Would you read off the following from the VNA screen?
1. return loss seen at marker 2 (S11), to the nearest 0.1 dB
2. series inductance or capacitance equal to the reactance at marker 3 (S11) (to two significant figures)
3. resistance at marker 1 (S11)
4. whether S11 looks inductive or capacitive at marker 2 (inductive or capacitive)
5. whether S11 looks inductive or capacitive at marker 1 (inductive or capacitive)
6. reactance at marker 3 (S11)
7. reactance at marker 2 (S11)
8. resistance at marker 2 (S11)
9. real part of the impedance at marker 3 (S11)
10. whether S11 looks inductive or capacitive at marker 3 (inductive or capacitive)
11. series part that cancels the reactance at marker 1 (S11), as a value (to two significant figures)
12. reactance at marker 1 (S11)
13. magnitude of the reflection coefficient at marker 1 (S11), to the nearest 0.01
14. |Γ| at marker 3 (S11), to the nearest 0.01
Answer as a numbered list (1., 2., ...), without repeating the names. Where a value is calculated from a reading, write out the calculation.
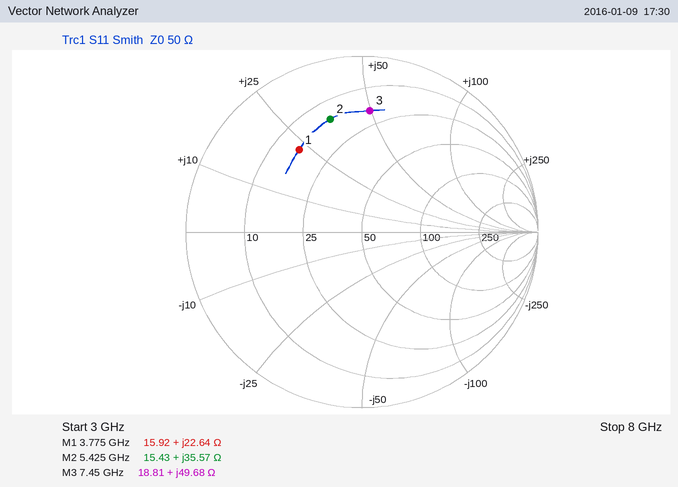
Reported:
1. 3.5 dB
2. L = 49.68 Ω/(2π × 7.45 GHz) ≈ 1.1 nH
3. 15.92 Ω
4. inductive
5. inductive
6. +49.68 Ω
7. +35.57 Ω
8. 15.43 Ω
9. 18.81 Ω
10. inductive
11. C = 1/(2π × 3.775 GHz × 22.64 Ω) ≈ 1.9 pF
12. +22.64 Ω
13. 0.59
14. 0.69
